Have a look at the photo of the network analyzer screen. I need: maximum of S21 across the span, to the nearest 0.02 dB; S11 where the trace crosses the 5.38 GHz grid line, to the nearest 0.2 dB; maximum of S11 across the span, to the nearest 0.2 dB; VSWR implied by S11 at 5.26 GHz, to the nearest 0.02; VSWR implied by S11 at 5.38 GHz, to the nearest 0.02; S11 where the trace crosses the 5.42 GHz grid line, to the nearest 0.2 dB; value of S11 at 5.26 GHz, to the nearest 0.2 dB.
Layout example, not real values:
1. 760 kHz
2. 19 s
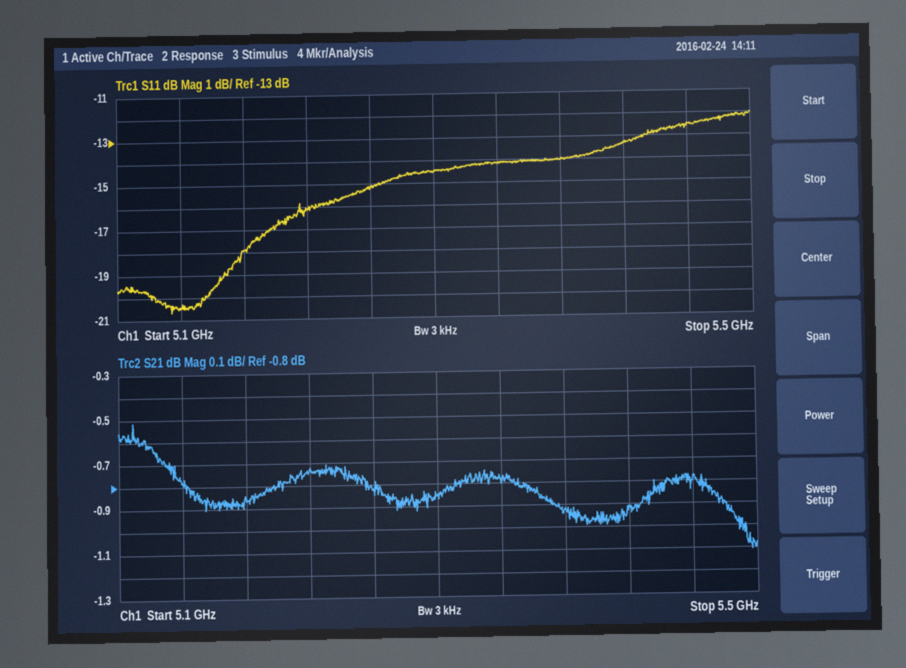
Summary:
1. -0.52 dB
2. -14.0 dB
3. -12.0 dB
4. 1.42
5. 1.50
6. -13.4 dB
7. -15.2 dB
